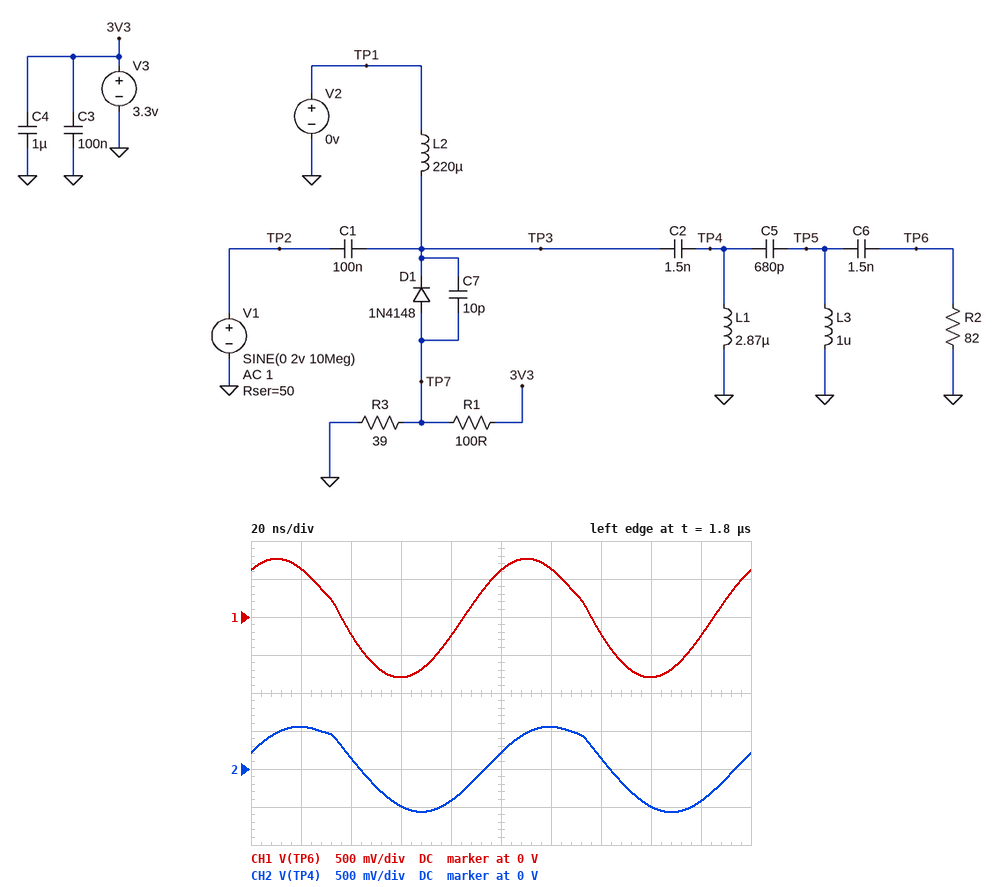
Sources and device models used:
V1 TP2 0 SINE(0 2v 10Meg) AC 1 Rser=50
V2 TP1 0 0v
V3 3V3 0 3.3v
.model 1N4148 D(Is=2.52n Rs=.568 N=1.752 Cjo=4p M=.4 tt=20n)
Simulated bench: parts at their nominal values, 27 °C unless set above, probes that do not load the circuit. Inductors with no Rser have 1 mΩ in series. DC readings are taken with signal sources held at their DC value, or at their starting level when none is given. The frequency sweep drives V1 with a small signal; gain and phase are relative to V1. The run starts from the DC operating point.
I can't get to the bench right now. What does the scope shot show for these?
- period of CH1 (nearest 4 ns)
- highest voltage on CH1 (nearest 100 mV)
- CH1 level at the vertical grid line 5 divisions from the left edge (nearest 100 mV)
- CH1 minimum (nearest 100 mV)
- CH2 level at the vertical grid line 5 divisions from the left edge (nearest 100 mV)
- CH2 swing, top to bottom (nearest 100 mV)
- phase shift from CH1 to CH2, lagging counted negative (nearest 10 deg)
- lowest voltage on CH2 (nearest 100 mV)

100 ns
800 mV
600 mV
-800 mV
200 mV
1.1 V
-30 deg
-600 mV
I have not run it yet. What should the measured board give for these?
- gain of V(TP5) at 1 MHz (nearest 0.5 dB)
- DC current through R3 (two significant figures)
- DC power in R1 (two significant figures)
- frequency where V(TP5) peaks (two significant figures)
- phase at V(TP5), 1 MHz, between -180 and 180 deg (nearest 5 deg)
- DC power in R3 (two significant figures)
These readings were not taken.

-52.0 dB
18 mA
68 mW
7.9 MHz
-15 deg
12 mW
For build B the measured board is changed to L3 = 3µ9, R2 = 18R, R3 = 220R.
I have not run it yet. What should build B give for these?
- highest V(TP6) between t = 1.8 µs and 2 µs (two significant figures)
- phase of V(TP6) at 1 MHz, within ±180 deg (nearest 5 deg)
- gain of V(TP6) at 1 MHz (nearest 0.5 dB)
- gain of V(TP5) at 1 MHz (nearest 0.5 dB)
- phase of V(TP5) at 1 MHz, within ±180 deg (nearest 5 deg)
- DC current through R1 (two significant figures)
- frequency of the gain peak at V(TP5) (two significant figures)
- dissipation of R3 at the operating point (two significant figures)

360 mV
60 deg
-49.5 dB
-34.0 dB
-20 deg
26 mA
1.7 MHz
2.5 mW
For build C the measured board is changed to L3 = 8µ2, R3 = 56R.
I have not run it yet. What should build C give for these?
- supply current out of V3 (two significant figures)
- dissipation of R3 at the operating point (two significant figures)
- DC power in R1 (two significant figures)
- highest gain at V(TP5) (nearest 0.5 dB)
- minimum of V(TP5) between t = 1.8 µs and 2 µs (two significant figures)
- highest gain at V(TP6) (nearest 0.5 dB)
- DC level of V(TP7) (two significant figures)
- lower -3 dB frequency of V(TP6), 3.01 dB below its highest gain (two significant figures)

26 mA
9.0 mW
67 mW
-6.5 dB
-690 mV
-7.5 dB
710 mV
1.7 MHz
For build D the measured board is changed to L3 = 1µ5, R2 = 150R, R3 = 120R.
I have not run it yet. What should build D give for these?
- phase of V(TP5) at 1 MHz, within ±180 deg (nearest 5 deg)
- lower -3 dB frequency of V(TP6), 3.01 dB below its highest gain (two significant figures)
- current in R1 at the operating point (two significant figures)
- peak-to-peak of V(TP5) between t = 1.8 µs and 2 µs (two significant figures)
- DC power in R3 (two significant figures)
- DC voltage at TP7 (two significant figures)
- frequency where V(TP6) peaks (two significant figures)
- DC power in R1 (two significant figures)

-20 deg
4.2 MHz
26 mA
2.2 V
4.4 mW
730 mV
6.5 MHz
66 mW
